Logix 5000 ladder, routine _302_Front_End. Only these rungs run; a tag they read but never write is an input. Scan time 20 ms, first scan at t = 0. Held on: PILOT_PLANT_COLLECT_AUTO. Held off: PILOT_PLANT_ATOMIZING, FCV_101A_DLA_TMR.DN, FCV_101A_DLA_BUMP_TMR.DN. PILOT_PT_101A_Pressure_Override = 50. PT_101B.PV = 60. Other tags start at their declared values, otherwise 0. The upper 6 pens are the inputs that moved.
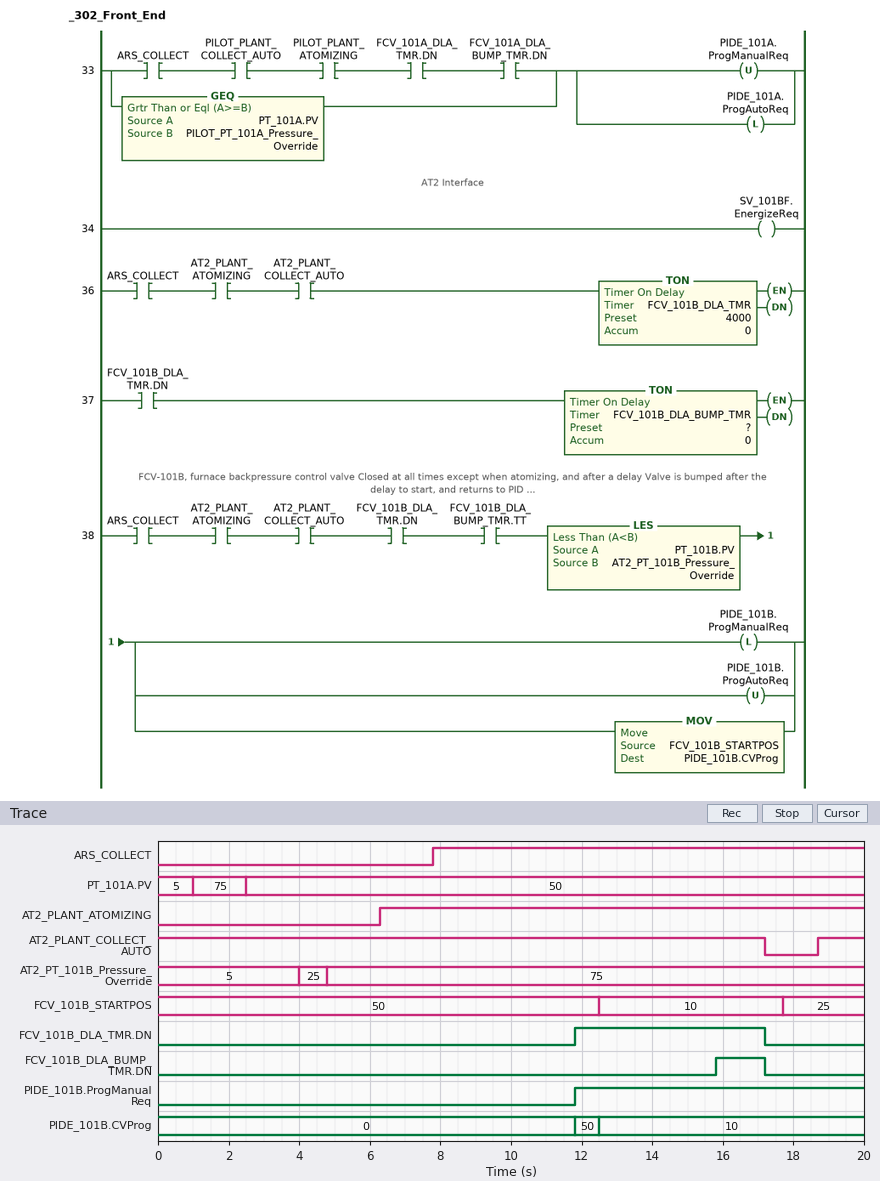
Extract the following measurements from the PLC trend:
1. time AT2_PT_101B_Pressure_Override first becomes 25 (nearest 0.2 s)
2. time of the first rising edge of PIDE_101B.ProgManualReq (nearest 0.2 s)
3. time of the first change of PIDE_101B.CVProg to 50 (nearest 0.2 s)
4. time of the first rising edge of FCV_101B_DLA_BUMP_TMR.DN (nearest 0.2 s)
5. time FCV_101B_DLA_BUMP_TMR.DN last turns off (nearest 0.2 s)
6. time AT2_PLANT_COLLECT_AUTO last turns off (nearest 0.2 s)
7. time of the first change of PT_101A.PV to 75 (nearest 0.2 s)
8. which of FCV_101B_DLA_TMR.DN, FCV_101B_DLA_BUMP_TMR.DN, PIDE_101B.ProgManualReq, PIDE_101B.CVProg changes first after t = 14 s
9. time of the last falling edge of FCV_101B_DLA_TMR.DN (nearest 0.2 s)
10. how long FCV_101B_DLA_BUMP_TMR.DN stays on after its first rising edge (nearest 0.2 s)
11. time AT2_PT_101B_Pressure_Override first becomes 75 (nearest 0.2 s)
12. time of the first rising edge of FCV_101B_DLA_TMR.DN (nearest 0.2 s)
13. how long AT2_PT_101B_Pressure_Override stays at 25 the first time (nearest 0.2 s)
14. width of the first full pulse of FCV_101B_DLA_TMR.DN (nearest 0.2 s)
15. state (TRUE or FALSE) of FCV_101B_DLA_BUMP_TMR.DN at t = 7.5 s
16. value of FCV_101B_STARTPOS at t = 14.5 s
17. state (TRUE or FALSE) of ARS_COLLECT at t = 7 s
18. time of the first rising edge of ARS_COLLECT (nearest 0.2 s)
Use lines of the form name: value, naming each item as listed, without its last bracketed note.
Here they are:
time AT2_PT_101B_Pressure_Override first becomes 25: 4.0 s
time of the first rising edge of PIDE_101B.ProgManualReq: 11.8 s
time of the first change of PIDE_101B.CVProg to 50: 11.8 s
time of the first rising edge of FCV_101B_DLA_BUMP_TMR.DN: 15.8 s
time FCV_101B_DLA_BUMP_TMR.DN last turns off: 17.2 s
time AT2_PLANT_COLLECT_AUTO last turns off: 17.2 s
time of the first change of PT_101A.PV to 75: 1.0 s
which of FCV_101B_DLA_TMR.DN, FCV_101B_DLA_BUMP_TMR.DN, PIDE_101B.ProgManualReq, PIDE_101B.CVProg changes first after t = 14 s: FCV_101B_DLA_BUMP_TMR.DN
time of the last falling edge of FCV_101B_DLA_TMR.DN: 17.2 s
how long FCV_101B_DLA_BUMP_TMR.DN stays on after its first rising edge: 1.4 s
time AT2_PT_101B_Pressure_Override first becomes 75: 4.8 s
time of the first rising edge of FCV_101B_DLA_TMR.DN: 11.8 s
how long AT2_PT_101B_Pressure_Override stays at 25 the first time: 0.8 s
width of the first full pulse of FCV_101B_DLA_TMR.DN: 5.4 s
state (TRUE or FALSE) of FCV_101B_DLA_BUMP_TMR.DN at t = 7.5 s: FALSE
value of FCV_101B_STARTPOS at t = 14.5 s: 10
state (TRUE or FALSE) of ARS_COLLECT at t = 7 s: FALSE
time of the first rising edge of ARS_COLLECT: 7.8 s
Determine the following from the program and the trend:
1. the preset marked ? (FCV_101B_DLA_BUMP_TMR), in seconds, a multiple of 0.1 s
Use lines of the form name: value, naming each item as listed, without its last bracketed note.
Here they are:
the preset marked ? (FCV_101B_DLA_BUMP_TMR), in seconds, a multiple of 0.1 s: 4.0 s
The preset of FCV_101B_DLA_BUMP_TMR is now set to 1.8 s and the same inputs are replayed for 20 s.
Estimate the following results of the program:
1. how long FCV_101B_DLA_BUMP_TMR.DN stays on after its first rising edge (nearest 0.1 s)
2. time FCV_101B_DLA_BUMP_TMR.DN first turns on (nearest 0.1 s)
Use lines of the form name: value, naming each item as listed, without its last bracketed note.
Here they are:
how long FCV_101B_DLA_BUMP_TMR.DN stays on after its first rising edge: 3.6 s
time FCV_101B_DLA_BUMP_TMR.DN first turns on: 13.6 s
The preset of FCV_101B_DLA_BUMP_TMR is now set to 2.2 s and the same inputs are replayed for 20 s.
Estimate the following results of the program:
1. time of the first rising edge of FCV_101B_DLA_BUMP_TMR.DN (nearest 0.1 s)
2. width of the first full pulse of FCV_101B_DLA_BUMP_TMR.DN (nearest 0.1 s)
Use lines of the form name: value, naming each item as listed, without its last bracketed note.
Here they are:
time of the first rising edge of FCV_101B_DLA_BUMP_TMR.DN: 14.0 s
width of the first full pulse of FCV_101B_DLA_BUMP_TMR.DN: 3.2 s
